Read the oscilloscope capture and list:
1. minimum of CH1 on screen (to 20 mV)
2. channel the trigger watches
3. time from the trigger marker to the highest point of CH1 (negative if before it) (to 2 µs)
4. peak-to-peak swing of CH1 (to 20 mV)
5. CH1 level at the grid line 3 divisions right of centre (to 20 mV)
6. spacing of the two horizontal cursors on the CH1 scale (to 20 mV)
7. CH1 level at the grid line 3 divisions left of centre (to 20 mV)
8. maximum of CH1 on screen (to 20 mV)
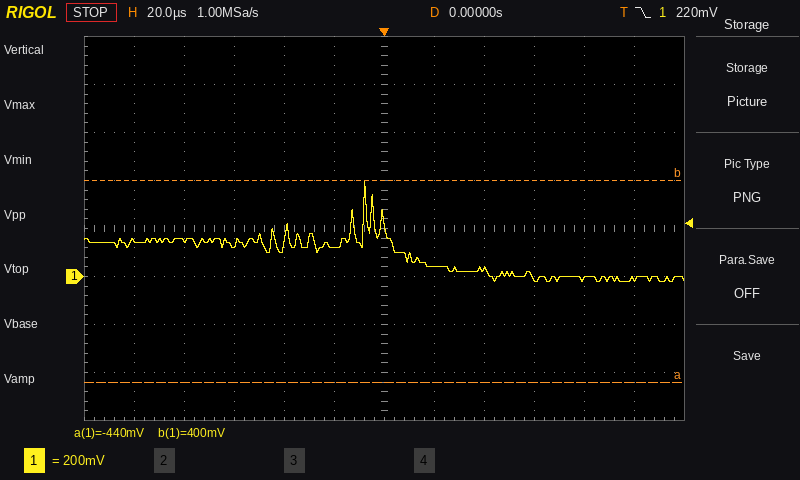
-20 mV
CH1
-8 µs
420 mV
0 mV
840 mV
140 mV
400 mV
